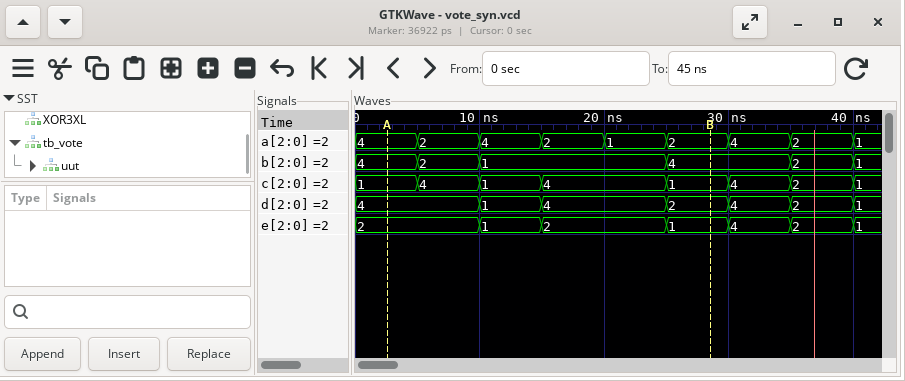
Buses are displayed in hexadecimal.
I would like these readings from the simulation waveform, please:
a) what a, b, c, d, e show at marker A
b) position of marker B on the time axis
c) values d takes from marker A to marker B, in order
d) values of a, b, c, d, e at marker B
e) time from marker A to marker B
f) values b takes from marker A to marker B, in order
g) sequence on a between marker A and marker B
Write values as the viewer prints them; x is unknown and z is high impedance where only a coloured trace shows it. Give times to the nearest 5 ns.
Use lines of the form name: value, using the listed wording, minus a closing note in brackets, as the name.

what a, b, c, d, e show at marker A: a=4, b=4, c=1, d=4, e=2
position of marker B on the time axis: 30 ns
values d takes from marker A to marker B, in order: 4, 1, 4, 2
values of a, b, c, d, e at marker B: a=2, b=4, c=1, d=2, e=1
time from marker A to marker B: 25 ns
values b takes from marker A to marker B, in order: 4, 2, 1, 4
sequence on a between marker A and marker B: 4, 2, 4, 2, 1, 2
